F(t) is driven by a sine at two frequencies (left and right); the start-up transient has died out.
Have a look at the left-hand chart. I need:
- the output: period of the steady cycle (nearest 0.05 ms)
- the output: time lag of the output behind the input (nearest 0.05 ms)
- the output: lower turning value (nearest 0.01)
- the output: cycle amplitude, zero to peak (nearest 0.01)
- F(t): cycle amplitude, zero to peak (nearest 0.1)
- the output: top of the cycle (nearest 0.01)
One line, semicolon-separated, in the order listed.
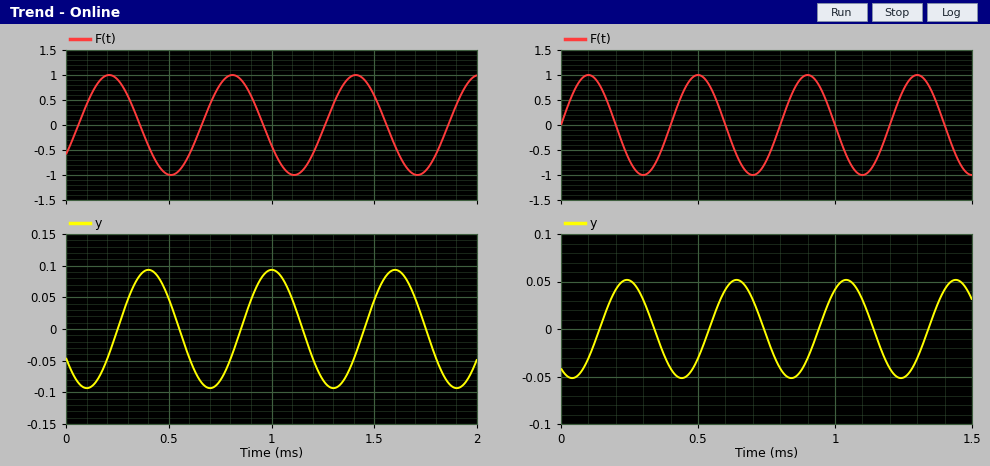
0.60 ms; 0.20 ms; -0.09; 0.09; 1.0; 0.09
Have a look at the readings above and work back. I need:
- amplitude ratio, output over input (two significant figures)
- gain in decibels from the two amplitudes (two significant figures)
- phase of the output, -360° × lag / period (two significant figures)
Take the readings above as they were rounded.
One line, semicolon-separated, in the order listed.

0.090; -21 dB; -120°
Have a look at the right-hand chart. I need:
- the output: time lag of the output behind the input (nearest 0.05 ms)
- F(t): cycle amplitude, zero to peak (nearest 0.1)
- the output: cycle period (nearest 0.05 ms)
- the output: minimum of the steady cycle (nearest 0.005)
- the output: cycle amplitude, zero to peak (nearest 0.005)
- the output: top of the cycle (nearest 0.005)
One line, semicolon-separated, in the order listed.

0.15 ms; 1.0; 0.40 ms; -0.050; 0.050; 0.050
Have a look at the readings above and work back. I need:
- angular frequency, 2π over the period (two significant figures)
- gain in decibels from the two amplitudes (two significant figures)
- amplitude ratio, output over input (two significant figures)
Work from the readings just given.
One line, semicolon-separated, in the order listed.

16 rad/ms; -26 dB; 0.050
